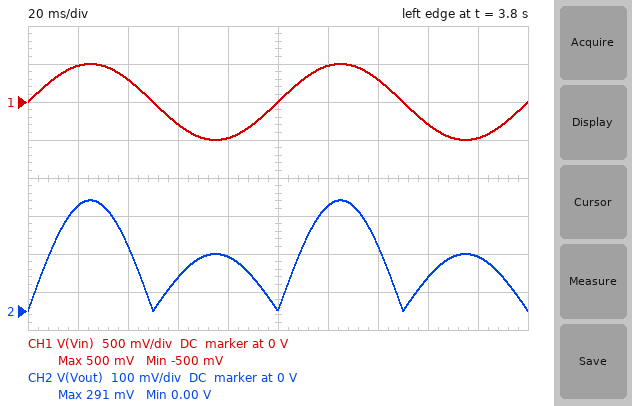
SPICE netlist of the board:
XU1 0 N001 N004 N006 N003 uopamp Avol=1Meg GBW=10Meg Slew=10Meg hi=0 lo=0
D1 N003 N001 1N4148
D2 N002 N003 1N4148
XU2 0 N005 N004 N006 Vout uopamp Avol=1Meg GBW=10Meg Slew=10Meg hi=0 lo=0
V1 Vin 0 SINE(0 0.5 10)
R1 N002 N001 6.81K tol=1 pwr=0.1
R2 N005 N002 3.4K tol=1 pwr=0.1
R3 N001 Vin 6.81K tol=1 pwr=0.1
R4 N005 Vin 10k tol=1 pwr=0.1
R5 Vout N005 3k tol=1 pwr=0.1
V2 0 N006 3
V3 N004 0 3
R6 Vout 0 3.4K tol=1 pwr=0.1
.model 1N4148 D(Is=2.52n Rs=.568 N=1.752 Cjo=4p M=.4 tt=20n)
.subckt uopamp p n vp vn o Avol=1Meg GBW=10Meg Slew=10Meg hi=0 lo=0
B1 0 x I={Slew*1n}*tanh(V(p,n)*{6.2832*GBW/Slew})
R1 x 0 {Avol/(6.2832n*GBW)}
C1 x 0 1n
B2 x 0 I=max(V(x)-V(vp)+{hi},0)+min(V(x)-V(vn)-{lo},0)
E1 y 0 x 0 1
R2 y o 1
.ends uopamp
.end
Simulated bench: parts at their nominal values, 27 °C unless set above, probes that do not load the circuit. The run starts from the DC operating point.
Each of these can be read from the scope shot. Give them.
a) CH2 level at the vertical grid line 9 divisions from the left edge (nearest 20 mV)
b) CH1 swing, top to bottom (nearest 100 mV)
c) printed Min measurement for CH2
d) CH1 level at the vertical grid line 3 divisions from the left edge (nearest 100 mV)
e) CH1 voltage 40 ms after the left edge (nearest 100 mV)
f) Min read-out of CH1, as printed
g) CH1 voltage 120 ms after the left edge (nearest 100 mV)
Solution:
140 mV
1.0 V
0.00 V
-300 mV
300 mV
-500 mV
500 mV
